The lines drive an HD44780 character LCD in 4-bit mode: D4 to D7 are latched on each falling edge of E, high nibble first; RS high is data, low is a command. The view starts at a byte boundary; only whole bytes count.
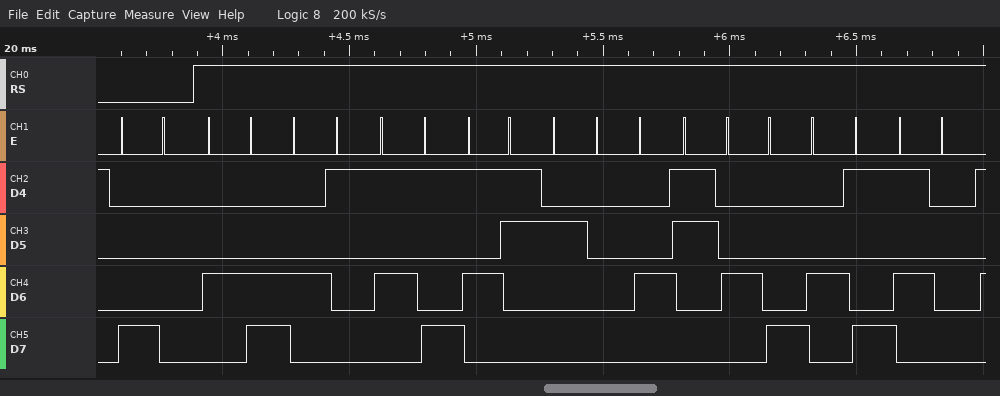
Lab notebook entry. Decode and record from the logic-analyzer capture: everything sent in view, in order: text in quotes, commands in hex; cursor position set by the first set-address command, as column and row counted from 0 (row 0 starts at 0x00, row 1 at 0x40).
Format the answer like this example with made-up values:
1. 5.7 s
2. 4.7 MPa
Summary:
1. 0x80 "LAYS CHIP"
2. column 0, row 0
